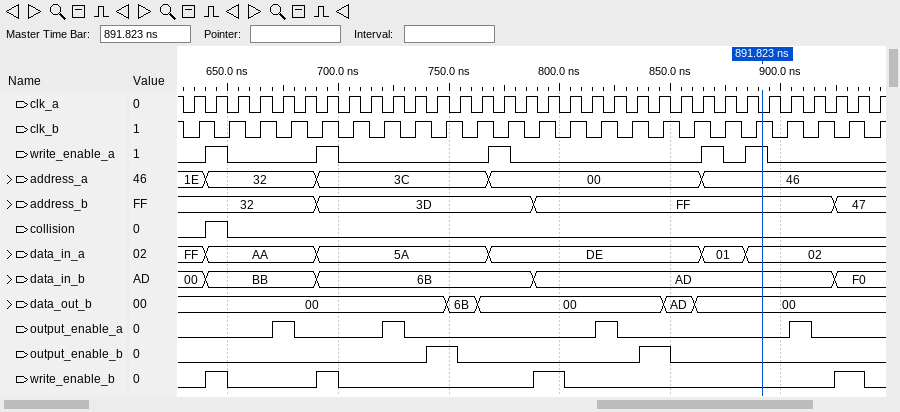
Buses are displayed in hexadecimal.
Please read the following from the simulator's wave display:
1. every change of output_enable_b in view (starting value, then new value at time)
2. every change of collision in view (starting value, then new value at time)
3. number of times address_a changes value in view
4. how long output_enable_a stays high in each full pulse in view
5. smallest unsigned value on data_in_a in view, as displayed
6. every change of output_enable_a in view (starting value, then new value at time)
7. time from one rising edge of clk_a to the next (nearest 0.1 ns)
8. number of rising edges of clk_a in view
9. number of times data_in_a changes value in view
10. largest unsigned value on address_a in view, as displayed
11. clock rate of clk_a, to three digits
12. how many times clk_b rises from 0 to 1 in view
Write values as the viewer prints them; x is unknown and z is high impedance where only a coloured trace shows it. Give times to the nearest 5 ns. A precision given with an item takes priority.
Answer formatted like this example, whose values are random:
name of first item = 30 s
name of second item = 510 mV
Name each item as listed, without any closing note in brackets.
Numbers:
every change of output_enable_b in view = 0, 1 at 740 ns, 0 at 755 ns, 1 at 835 ns, 0 at 850 ns
every change of collision in view = 0, 1 at 640 ns, 0 at 650 ns
number of times address_a changes value in view = 4
how long output_enable_a stays high in each full pulse in view = 10 ns, 10 ns, 10 ns, 10 ns
smallest unsigned value on data_in_a in view, as displayed = 01
every change of output_enable_a in view = 0, 1 at 670 ns, 0 at 680 ns, 1 at 720 ns, 0 at 730 ns, 1 at 815 ns, 0 at 825 ns, 1 at 905 ns, 0 at 915 ns
time from one rising edge of clk_a to the next = 10 ns
number of rising edges of clk_a in view = 32
number of times data_in_a changes value in view = 5
largest unsigned value on address_a in view, as displayed = 46
clock rate of clk_a, to three digits = 100 MHz
how many times clk_b rises from 0 to 1 in view = 23
